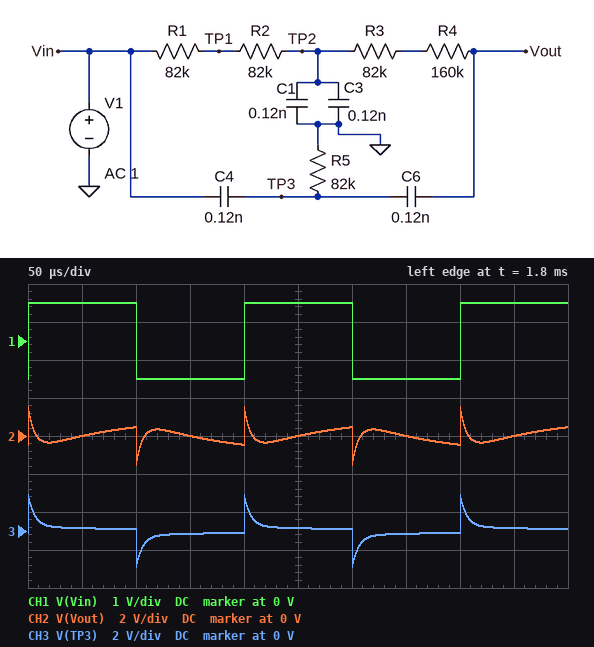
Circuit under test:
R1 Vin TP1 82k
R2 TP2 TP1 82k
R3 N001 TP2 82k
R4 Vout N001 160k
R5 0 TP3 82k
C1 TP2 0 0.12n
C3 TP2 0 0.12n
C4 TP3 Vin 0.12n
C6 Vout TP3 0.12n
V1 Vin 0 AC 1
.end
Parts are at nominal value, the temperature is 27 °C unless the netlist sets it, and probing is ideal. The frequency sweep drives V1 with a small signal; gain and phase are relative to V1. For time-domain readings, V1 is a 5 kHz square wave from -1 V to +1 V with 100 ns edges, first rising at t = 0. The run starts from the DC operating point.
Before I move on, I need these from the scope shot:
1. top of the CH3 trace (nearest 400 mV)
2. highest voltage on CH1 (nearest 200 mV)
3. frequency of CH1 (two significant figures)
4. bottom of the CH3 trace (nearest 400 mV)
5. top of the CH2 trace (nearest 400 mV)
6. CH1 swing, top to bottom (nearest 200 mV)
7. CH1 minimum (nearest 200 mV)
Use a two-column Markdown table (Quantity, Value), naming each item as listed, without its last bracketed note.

| Quantity | Value |
|---|---|
| top of the CH3 trace | 2.0 V |
| highest voltage on CH1 | 1.0 V |
| frequency of CH1 | 5.0 kHz |
| bottom of the CH3 trace | -2.0 V |
| top of the CH2 trace | 1.6 V |
| CH1 swing, top to bottom | 2.0 V |
| CH1 minimum | -1.0 V |
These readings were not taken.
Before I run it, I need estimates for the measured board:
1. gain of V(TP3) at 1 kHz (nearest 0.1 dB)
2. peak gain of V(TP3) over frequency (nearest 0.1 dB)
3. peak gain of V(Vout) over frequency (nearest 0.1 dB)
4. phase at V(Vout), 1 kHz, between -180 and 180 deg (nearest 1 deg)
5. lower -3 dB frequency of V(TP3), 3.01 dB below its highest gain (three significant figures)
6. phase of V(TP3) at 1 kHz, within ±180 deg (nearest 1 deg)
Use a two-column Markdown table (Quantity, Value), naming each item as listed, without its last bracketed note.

| Quantity | Value |
|---|---|
| gain of V(TP3) at 1 kHz | -19.1 dB |
| peak gain of V(TP3) over frequency | 0 dB |
| peak gain of V(Vout) over frequency | 0 dB |
| phase at V(Vout), 1 kHz, between -180 and 180 deg | -30 deg |
| lower -3 dB frequency of V(TP3), 3.01 dB below its highest gain | 24.4 kHz |
| phase of V(TP3) at 1 kHz, within ±180 deg | 69 deg |
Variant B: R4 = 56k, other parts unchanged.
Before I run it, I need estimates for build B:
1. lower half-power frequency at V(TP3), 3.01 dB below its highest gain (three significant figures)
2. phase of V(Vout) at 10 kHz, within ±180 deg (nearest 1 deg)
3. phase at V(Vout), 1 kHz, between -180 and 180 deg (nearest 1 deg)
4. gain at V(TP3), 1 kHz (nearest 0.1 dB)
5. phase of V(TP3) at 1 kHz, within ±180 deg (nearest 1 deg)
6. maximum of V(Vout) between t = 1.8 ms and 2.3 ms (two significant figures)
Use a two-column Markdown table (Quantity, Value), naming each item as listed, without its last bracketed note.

| Quantity | Value |
|---|---|
| lower half-power frequency at V(TP3), 3.01 dB below its highest gain | 30.3 kHz |
| phase of V(Vout) at 10 kHz, within ±180 deg | 77 deg |
| phase at V(Vout), 1 kHz, between -180 and 180 deg | -26 deg |
| gain at V(TP3), 1 kHz | -18.9 dB |
| phase of V(TP3) at 1 kHz, within ±180 deg | 71 deg |
| maximum of V(Vout) between t = 1.8 ms and 2.3 ms | 1.4 V |
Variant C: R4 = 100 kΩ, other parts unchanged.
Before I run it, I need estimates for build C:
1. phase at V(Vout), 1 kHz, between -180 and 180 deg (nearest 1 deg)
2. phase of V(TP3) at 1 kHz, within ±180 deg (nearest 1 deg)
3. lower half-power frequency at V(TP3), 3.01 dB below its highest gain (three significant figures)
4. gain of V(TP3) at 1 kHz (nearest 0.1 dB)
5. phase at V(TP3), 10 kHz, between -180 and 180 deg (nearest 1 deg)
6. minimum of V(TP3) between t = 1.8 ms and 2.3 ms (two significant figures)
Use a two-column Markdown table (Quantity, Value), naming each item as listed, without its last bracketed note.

| Quantity | Value |
|---|---|
| phase at V(Vout), 1 kHz, between -180 and 180 deg | -27 deg |
| phase of V(TP3) at 1 kHz, within ±180 deg | 70 deg |
| lower half-power frequency at V(TP3), 3.01 dB below its highest gain | 27.0 kHz |
| gain of V(TP3) at 1 kHz | -19.0 dB |
| phase at V(TP3), 10 kHz, between -180 and 180 deg | 46 deg |
| minimum of V(TP3) between t = 1.8 ms and 2.3 ms | -1.9 V |
